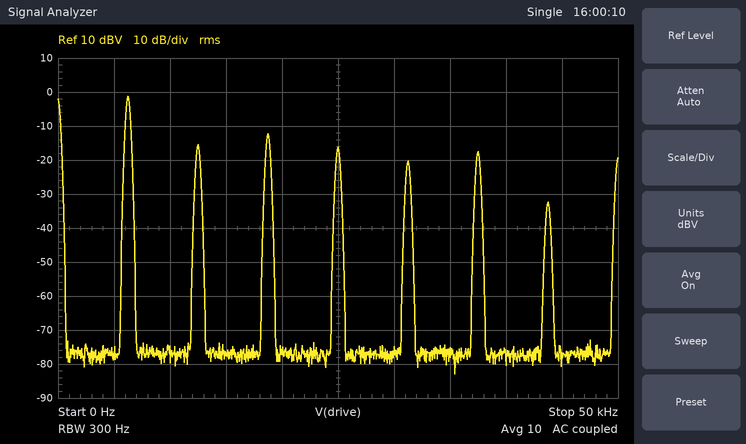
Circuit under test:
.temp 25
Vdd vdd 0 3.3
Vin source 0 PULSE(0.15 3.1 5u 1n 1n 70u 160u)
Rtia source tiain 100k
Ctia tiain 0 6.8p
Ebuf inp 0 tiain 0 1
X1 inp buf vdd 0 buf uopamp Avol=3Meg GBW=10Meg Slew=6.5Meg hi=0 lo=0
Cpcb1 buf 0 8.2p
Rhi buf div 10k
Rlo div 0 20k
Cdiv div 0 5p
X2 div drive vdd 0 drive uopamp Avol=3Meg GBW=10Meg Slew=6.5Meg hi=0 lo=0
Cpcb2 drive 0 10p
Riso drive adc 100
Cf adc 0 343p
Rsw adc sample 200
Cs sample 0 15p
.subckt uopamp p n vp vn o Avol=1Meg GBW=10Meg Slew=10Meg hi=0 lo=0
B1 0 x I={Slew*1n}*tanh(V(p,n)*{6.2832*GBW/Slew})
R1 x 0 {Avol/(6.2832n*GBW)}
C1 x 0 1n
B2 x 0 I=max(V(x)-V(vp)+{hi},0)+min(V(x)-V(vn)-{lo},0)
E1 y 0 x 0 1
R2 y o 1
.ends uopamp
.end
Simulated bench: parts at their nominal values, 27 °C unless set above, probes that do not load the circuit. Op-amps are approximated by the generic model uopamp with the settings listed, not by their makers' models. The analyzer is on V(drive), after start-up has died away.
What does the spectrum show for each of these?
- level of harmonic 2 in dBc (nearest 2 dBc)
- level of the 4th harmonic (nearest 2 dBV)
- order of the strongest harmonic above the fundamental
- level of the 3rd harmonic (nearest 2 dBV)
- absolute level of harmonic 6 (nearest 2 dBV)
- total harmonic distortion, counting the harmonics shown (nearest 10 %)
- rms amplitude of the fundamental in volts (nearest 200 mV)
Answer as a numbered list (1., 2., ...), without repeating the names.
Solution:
1. -14 dBc
2. -16 dBV
3. 3
4. -12 dBV
5. -18 dBV
6. 40 %
7. 800 mV
